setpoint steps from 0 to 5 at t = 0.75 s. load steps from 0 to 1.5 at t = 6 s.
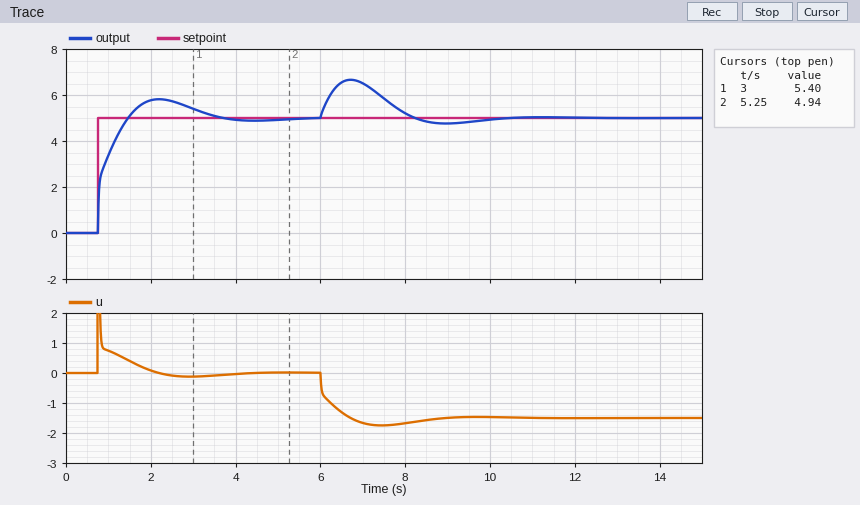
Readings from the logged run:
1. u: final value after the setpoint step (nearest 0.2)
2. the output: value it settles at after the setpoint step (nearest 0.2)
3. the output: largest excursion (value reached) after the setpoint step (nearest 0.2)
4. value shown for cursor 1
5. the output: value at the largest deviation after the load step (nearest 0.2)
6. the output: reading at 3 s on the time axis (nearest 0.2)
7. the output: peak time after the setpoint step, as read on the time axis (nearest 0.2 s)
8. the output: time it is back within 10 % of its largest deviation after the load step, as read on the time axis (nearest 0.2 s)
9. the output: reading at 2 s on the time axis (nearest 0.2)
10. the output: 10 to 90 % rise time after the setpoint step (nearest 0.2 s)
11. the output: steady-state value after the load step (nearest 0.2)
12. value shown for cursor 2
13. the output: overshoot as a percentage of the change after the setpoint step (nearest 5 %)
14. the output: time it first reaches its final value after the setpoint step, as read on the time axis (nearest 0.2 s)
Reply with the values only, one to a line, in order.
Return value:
0.0
5.0
5.8
5.40
6.6
5.4
2.2 s
9.6 s
5.8
0.6 s
5.0
4.94
15 %
1.4 s
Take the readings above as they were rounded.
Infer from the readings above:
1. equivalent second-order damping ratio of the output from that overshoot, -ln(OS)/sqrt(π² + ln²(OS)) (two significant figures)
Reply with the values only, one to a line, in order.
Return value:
0.52
